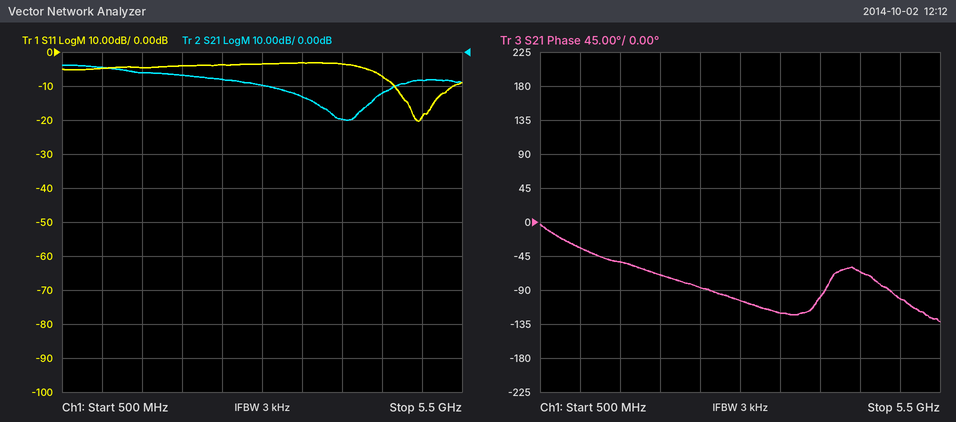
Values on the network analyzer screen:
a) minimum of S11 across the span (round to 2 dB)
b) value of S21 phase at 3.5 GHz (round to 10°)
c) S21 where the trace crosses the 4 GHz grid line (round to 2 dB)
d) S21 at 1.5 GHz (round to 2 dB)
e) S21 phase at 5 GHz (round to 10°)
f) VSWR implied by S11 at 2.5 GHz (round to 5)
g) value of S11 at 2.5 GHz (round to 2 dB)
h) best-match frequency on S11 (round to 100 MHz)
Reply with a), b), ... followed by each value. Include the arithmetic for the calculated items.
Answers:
a) -20 dB
b) -120°
c) -20 dB
d) -6 dB
e) -100°
f) |Γ| = 10^(-4/20) = 0.6310; VSWR = (1 + 0.6310)/(1 − 0.6310) ≈ 4.42, so 5 to the nearest 5
g) -4 dB
h) 5.0 GHz
